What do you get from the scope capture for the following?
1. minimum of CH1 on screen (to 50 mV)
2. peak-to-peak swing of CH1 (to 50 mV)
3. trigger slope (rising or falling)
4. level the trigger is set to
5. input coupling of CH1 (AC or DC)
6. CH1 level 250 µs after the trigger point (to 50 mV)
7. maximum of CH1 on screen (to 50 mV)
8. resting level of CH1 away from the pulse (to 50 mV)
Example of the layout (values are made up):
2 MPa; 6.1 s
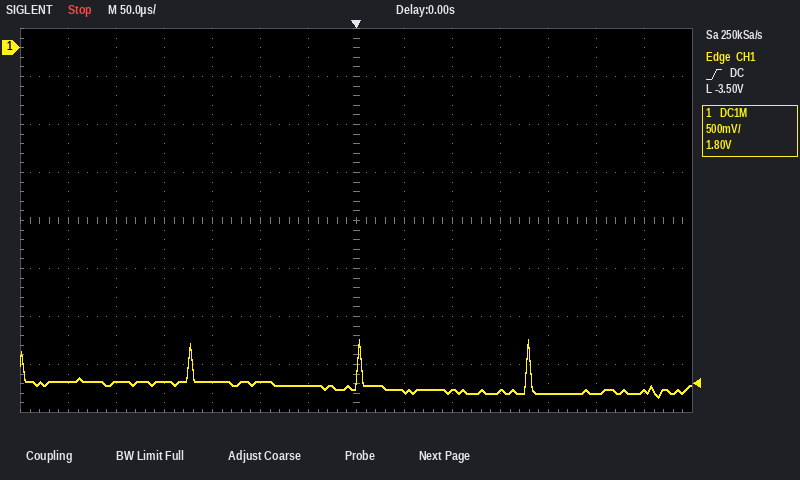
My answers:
-3.65 V; 600 mV; rising; -3.50 V; DC; -3.60 V; -3.05 V; -3.50 V
